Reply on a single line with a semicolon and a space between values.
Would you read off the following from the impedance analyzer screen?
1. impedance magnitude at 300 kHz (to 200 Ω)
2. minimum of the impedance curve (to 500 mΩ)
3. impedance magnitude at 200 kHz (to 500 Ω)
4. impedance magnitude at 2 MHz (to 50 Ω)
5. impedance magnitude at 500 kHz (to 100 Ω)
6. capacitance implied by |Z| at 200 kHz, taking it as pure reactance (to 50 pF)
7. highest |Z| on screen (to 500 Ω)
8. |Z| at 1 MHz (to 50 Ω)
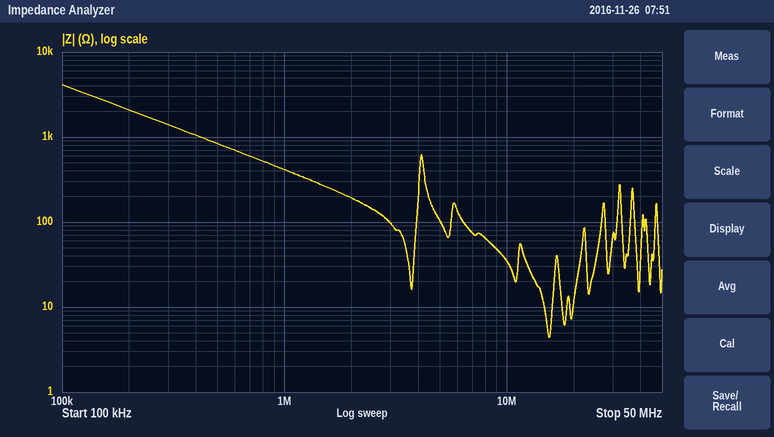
1.4 kΩ; 4.5 Ω; 2.0 kΩ; 200 Ω; 800 Ω; 400 pF; 4.0 kΩ; 400 Ω
